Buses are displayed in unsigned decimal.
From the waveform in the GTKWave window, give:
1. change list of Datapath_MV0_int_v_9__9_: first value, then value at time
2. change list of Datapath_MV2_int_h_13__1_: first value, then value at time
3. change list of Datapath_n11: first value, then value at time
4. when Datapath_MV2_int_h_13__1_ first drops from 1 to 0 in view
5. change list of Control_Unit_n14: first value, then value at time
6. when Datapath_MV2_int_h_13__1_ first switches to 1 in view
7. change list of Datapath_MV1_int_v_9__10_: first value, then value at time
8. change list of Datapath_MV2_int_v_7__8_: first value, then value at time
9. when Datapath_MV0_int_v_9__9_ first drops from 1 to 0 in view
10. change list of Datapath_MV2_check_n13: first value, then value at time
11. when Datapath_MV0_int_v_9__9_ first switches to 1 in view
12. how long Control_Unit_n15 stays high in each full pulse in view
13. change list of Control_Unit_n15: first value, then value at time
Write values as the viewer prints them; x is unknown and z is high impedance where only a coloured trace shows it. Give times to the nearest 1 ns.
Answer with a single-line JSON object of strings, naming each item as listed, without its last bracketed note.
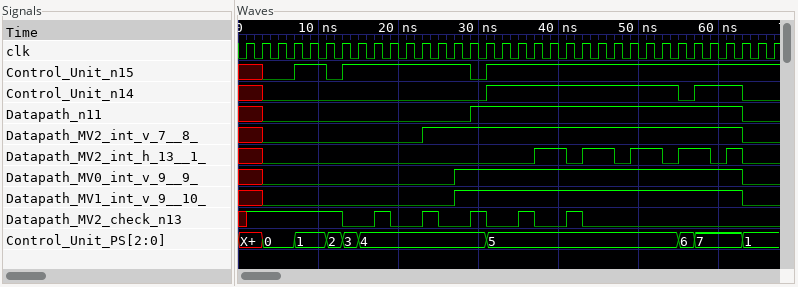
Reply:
{"change list of Datapath_MV0_int_v_9__9_: first value, then value at time": "x, 0 at 3 ns, 1 at 27 ns, 0 at 63 ns", "change list of Datapath_MV2_int_h_13__1_: first value, then value at time": "x, 0 at 3 ns, 1 at 37 ns, 0 at 41 ns, 1 at 43 ns, 0 at 47 ns, 1 at 49 ns, 0 at 53 ns, 1 at 55 ns, 0 at 59 ns, 1 at 61 ns, 0 at 63 ns", "change list of Datapath_n11: first value, then value at time": "x, 0 at 3 ns, 1 at 29 ns, 0 at 63 ns", "when Datapath_MV2_int_h_13__1_ first drops from 1 to 0 in view": "41 ns", "change list of Control_Unit_n14: first value, then value at time": "x, 0 at 3 ns, 1 at 31 ns, 0 at 55 ns, 1 at 57 ns, 0 at 63 ns", "when Datapath_MV2_int_h_13__1_ first switches to 1 in view": "37 ns", "change list of Datapath_MV1_int_v_9__10_: first value, then value at time": "x, 0 at 3 ns, 1 at 27 ns, 0 at 63 ns", "change list of Datapath_MV2_int_v_7__8_: first value, then value at time": "x, 0 at 3 ns, 1 at 23 ns, 0 at 63 ns", "when Datapath_MV0_int_v_9__9_ first drops from 1 to 0 in view": "63 ns", "change list of Datapath_MV2_check_n13: first value, then value at time": "x, 1 at 1 ns, 0 at 13 ns, 1 at 17 ns, 0 at 19 ns, 1 at 23 ns, 0 at 25 ns, 1 at 29 ns, 0 at 31 ns, 1 at 35 ns, 0 at 37 ns, 1 at 41 ns, 0 at 43 ns", "when Datapath_MV0_int_v_9__9_ first switches to 1 in view": "27 ns", "how long Control_Unit_n15 stays high in each full pulse in view": "4 ns, 16 ns", "change list of Control_Unit_n15: first value, then value at time": "x, 0 at 3 ns, 1 at 7 ns, 0 at 11 ns, 1 at 13 ns, 0 at 29 ns, 1 at 31 ns"}
